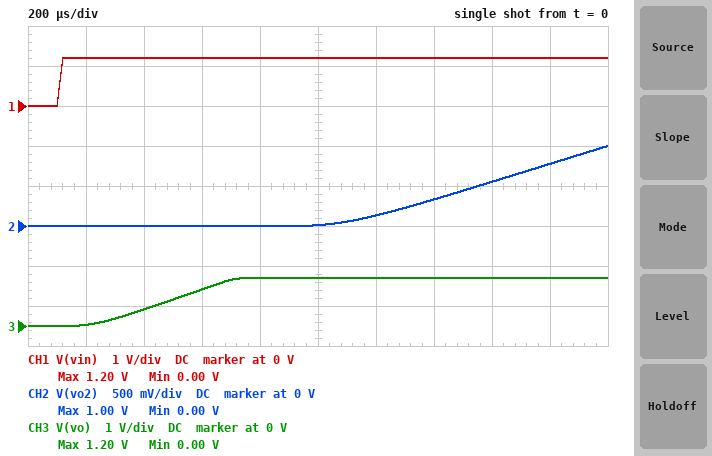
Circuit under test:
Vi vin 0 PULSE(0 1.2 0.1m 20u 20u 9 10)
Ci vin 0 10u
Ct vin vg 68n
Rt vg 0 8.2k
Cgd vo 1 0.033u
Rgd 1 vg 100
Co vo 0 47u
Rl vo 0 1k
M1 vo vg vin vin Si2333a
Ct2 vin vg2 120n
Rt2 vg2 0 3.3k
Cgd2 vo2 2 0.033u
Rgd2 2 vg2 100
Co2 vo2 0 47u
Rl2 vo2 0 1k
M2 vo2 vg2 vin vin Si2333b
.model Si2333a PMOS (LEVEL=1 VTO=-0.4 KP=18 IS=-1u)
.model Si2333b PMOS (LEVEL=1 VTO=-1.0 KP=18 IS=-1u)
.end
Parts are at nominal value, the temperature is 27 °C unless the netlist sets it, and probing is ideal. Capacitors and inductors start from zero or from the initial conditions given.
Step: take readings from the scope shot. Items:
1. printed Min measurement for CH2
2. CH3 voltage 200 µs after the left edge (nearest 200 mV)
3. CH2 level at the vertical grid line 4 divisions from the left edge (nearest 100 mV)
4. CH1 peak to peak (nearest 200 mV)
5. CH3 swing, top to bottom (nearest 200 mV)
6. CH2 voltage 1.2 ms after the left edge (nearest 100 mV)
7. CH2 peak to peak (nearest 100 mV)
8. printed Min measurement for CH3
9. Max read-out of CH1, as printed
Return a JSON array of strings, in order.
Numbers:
["0.00 V", "0 V", "0 V", "1.2 V", "1.2 V", "100 mV", "1.0 V", "0.00 V", "1.20 V"]
